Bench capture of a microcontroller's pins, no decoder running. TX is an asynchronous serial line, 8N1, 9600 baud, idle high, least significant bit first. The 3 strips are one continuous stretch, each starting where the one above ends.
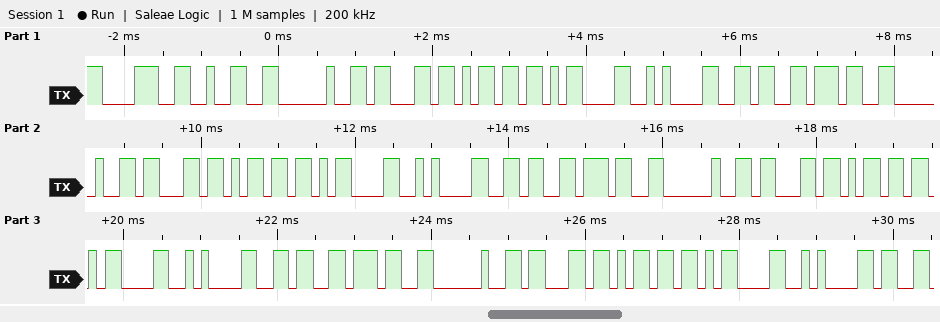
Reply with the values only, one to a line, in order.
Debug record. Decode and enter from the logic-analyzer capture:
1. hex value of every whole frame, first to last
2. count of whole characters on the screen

38 32 20 63 6D 0D 0A 36 37 20 63 6D 0D 0A 36 37 20 63 6D 0D 0A 36 37 20 63 6D 0D 0A
28
